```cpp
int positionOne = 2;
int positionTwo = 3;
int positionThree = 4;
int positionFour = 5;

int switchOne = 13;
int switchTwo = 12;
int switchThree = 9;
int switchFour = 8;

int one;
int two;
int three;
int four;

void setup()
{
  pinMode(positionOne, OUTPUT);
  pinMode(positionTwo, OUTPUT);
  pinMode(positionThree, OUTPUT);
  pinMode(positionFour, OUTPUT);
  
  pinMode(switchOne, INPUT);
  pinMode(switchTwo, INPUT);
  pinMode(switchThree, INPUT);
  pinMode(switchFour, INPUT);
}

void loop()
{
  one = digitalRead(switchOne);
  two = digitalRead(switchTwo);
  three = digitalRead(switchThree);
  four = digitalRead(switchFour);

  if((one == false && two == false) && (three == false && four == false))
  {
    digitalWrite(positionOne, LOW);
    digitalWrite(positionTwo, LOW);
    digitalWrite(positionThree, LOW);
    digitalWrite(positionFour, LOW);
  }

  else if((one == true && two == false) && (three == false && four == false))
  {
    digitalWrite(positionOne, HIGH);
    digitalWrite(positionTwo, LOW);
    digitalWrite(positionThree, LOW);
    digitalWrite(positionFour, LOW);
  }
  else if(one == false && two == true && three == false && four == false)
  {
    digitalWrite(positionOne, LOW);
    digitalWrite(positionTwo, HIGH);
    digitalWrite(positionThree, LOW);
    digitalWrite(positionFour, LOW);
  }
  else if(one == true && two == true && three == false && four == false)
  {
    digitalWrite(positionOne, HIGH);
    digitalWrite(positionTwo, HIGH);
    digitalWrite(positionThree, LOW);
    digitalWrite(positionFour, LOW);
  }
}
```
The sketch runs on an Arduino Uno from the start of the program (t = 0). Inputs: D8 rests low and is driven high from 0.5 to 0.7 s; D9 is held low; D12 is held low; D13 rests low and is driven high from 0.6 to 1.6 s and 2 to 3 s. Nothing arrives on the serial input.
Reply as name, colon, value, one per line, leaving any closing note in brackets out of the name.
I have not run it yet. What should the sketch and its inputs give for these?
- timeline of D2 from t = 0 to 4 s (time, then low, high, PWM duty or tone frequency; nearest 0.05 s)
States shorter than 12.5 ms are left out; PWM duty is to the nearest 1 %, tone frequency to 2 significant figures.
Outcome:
timeline of D2 from t = 0 to 4 s: 0 s low; 0.7 s high; 1.6 s low; 2 s high; 3 s low
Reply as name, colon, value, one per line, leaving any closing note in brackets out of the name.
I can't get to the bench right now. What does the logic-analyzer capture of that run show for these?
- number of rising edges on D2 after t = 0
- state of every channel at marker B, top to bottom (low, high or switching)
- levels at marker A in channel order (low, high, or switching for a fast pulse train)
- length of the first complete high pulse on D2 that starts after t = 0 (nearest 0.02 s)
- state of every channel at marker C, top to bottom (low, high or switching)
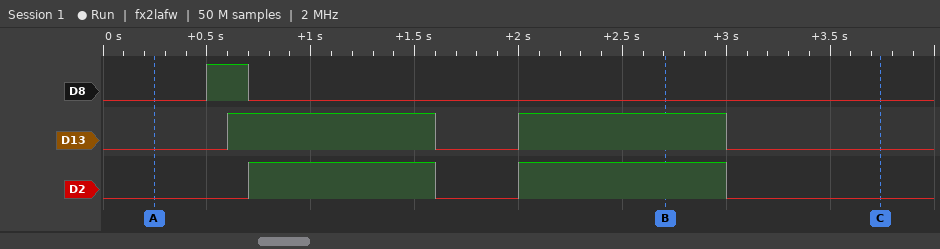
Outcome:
number of rising edges on D2 after t = 0: 2
state of every channel at marker B, top to bottom: D8 low, D13 high, D2 high
levels at marker A in channel order: D8 low, D13 low, D2 low
length of the first complete high pulse on D2 that starts after t = 0: 0.90 s
state of every channel at marker C, top to bottom: D8 low, D13 low, D2 low
